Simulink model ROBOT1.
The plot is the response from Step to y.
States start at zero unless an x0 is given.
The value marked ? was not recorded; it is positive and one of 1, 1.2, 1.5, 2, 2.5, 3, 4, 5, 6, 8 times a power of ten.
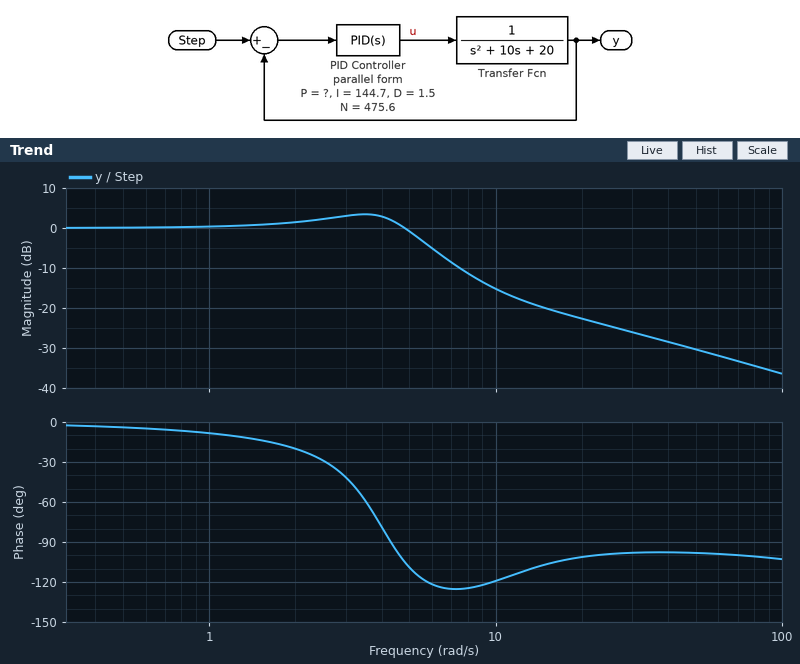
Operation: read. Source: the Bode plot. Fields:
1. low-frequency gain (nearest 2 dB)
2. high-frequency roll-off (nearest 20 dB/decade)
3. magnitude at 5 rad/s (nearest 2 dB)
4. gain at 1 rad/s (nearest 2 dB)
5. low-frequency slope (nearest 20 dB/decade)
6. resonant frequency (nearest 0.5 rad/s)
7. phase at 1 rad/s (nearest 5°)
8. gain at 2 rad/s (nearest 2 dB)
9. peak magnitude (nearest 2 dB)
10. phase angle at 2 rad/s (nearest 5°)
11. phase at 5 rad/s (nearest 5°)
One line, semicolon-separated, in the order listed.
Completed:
0 dB; -20 dB/decade; 0 dB; 0 dB; 0 dB/decade; 3.5 rad/s; -10°; 2 dB; 4 dB; -20°; -110°
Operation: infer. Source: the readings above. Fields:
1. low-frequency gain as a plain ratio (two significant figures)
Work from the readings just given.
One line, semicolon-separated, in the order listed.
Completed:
1.0
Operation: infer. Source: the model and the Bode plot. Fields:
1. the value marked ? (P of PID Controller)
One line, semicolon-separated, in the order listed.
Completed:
20
